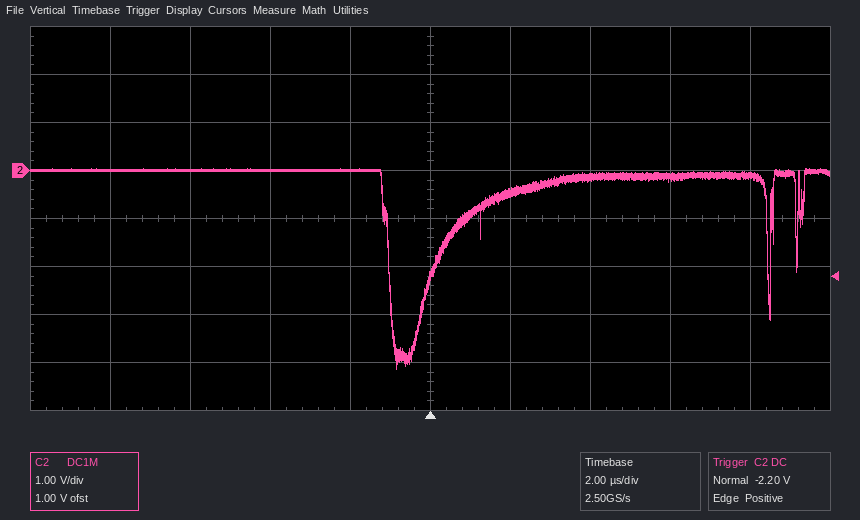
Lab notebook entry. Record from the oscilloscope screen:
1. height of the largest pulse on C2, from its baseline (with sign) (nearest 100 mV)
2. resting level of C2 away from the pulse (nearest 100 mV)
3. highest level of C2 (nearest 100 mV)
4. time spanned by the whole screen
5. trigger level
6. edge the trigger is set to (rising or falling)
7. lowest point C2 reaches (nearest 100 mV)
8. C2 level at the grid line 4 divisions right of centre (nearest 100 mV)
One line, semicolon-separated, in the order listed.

-4.1 V; 0.0 V; 0.0 V; 20 µs; -2.20 V; rising; -4.1 V; -100 mV
